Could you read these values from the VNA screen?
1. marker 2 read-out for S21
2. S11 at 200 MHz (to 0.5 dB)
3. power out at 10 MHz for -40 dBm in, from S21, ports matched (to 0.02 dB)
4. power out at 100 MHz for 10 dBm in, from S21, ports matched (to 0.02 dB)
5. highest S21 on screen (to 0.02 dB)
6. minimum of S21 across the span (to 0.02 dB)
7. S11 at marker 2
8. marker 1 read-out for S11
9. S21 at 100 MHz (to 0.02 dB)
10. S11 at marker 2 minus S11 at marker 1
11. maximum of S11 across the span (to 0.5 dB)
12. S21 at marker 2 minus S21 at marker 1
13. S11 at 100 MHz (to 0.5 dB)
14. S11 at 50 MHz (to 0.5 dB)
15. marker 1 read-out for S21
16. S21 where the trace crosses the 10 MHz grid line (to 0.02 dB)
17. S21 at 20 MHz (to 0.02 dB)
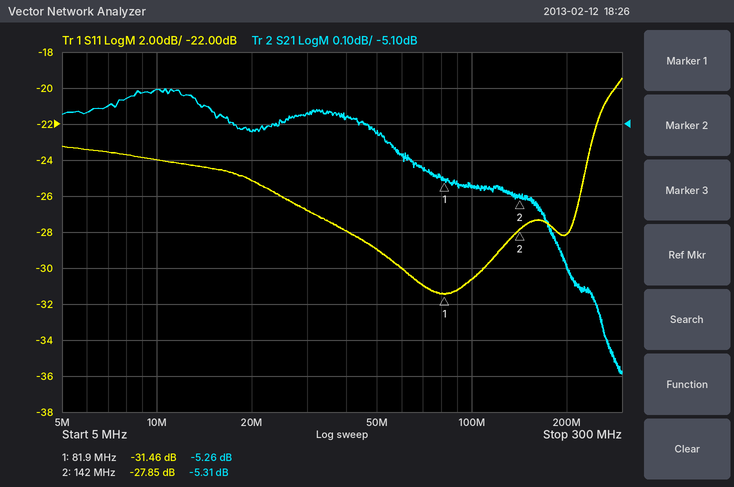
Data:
-5.31 dB
-28.0 dB
-45.00 dBm
4.72 dBm
-5.00 dB
-5.80 dB
-27.85 dB
-31.46 dB
-5.28 dB
3.61 dB
-19.5 dB
-0.05 dB
-30.5 dB
-29.0 dB
-5.26 dB
-5.00 dB
-5.12 dB
